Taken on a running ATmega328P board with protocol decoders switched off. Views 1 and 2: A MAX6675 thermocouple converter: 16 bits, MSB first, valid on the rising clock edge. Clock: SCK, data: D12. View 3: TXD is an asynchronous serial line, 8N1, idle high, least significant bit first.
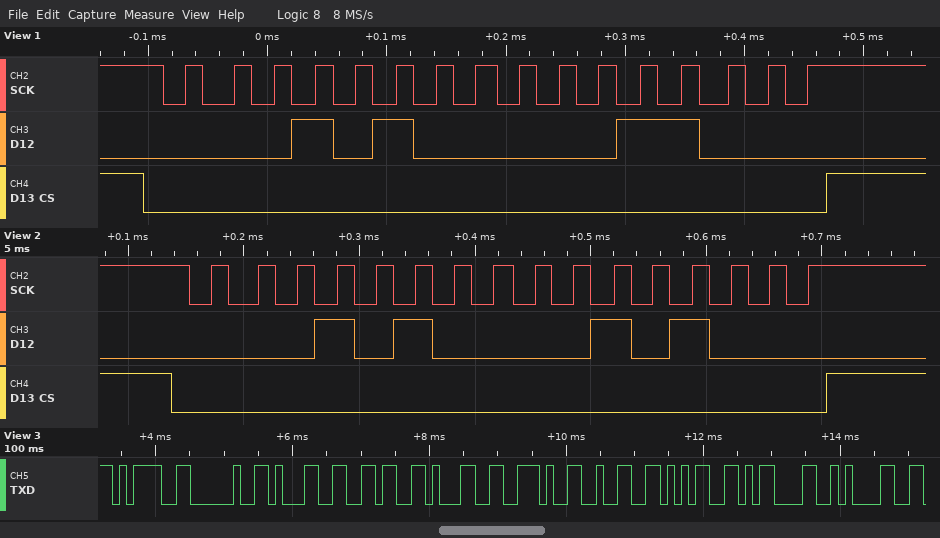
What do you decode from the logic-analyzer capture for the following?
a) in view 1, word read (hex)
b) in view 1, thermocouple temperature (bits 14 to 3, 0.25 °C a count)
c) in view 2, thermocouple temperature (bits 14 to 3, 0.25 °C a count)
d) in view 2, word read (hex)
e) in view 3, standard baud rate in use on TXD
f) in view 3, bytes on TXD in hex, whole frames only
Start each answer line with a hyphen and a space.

- 0x1418
- 160.75 °C
- 161.25 °C
- 0x1428
- 9600 baud
- 3D 20 31 36 31 2E 32 35 0D 0A
